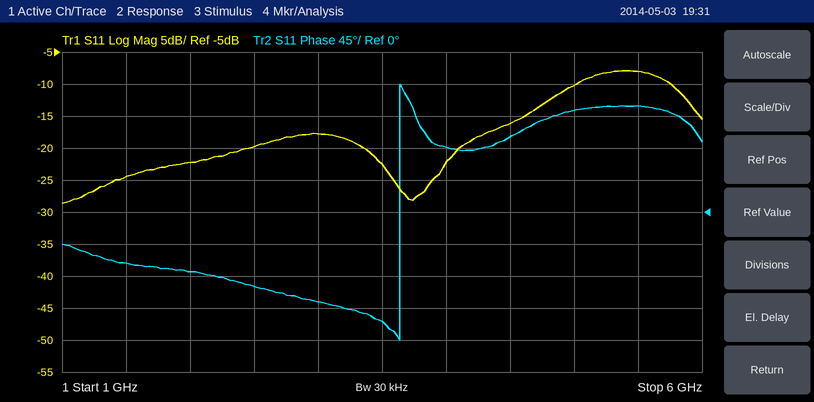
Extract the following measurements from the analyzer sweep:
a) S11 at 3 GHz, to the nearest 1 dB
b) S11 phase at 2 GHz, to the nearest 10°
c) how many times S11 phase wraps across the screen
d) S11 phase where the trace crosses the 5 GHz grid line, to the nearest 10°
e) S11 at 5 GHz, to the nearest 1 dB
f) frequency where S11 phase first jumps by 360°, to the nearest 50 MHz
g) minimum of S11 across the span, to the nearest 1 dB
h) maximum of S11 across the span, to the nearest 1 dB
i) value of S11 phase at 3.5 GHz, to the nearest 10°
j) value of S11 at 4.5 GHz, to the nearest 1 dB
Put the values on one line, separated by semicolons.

-18 dB; -80°; 1; 140°; -10 dB; 3.65 GHz; -29 dB; -8 dB; -150°; -16 dB
